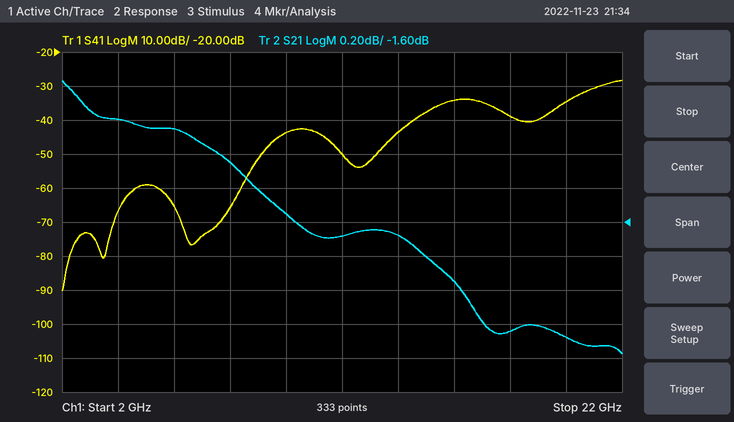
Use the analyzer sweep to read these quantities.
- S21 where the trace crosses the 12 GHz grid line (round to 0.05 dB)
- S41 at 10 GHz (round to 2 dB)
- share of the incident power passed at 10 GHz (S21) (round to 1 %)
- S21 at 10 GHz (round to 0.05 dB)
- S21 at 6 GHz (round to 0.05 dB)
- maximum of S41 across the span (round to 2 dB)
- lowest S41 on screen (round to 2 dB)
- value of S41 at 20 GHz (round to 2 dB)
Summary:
-1.70 dB
-44 dB
70 %
-1.55 dB
-1.05 dB
-28 dB
-90 dB
-34 dB
